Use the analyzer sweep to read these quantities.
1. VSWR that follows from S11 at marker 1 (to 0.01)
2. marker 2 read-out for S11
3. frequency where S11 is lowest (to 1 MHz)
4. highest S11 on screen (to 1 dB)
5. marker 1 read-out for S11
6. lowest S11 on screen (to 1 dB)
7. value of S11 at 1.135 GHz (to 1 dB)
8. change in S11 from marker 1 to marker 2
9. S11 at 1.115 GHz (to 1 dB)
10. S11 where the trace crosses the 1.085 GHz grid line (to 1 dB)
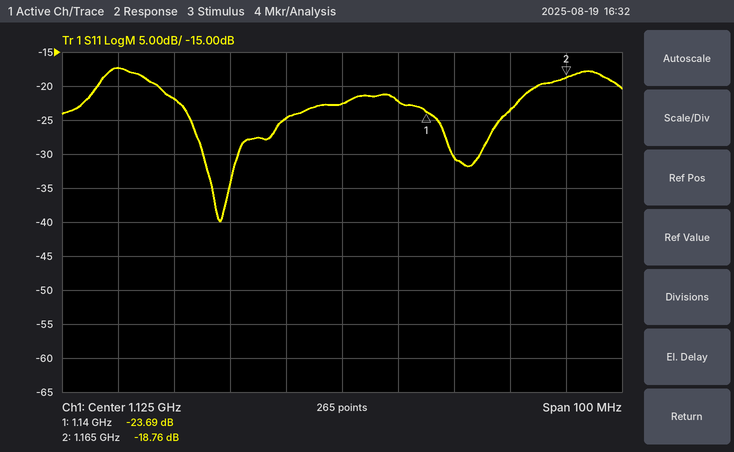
1.14
-18.76 dB
1.103 GHz
-17 dB
-23.69 dB
-40 dB
-22 dB
4.93 dB
-25 dB
-17 dB
